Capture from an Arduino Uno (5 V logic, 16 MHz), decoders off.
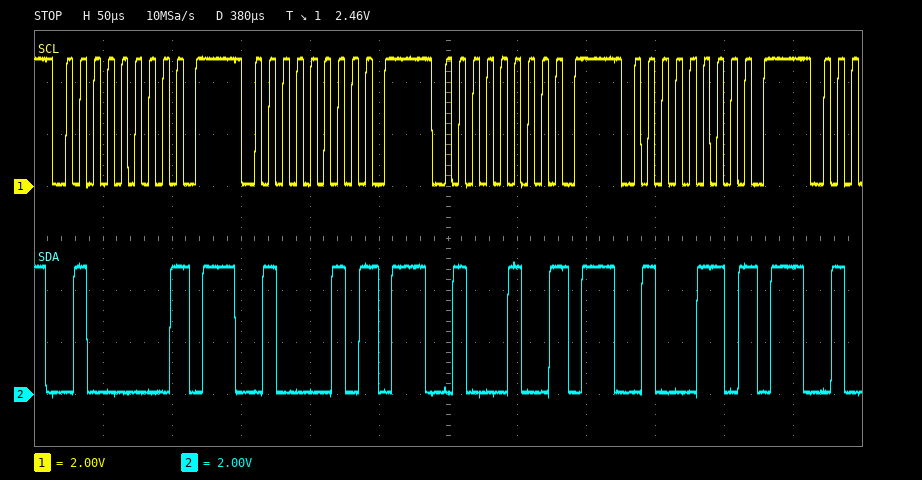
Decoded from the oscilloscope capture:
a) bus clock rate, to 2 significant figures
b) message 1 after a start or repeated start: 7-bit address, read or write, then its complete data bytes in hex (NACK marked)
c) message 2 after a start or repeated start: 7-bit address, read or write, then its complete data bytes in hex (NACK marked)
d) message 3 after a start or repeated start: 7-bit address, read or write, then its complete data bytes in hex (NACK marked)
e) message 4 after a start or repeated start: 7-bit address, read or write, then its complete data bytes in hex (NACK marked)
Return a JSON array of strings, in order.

["100 kHz", "0x20 write NACK", "0x21 write NACK", "0x22 write NACK", "0x23 write NACK"]
